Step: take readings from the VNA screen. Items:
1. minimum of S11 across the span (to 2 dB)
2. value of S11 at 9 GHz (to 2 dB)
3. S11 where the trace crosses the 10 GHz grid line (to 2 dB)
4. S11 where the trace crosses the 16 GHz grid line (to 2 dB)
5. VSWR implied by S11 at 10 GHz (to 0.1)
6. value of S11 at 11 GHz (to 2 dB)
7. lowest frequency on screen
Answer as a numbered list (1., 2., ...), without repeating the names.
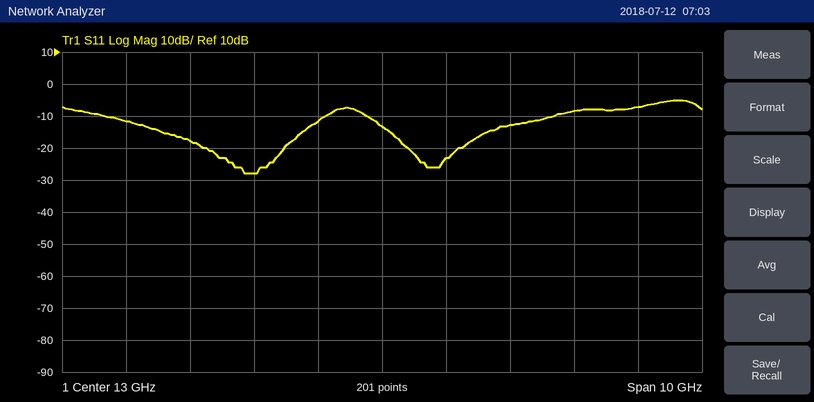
1. -28 dB
2. -12 dB
3. -18 dB
4. -8 dB
5. 1.3
6. -28 dB
7. 8 GHz
